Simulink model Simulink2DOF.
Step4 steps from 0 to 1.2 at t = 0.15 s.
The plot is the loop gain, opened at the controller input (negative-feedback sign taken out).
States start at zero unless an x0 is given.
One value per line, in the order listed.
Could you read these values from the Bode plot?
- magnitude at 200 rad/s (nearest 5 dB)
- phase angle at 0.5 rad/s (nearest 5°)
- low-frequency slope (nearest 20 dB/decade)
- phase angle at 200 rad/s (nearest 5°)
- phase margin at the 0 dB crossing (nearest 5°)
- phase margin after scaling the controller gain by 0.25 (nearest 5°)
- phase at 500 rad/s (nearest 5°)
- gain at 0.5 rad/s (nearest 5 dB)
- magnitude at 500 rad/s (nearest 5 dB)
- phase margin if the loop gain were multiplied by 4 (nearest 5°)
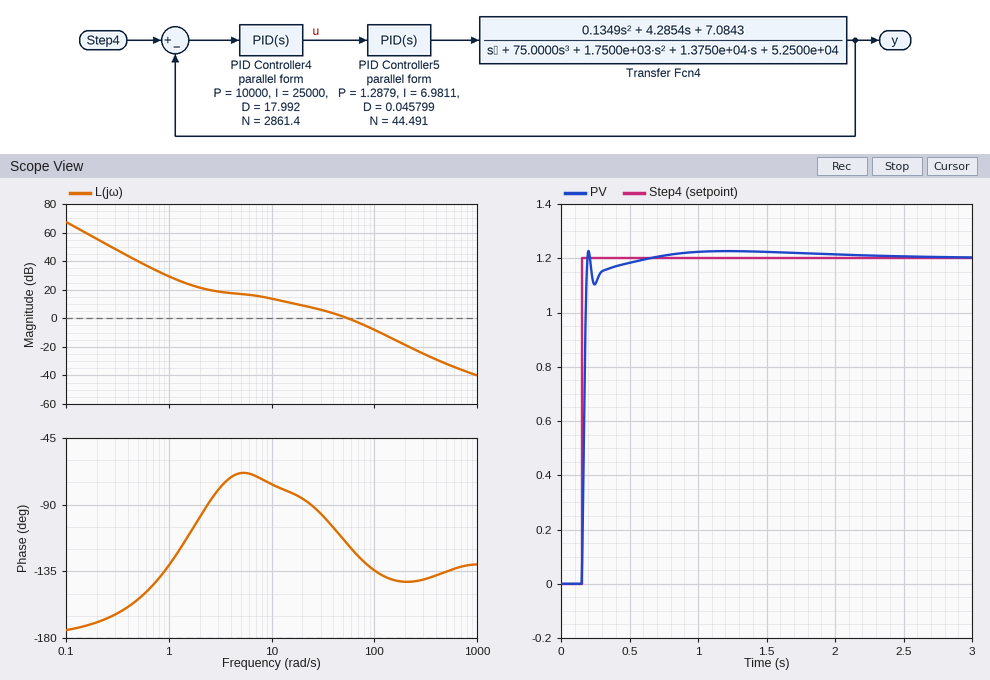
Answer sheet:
-20 dB
-155°
-40 dB/decade
-140°
65°
100°
-135°
40 dB
-30 dB
40°
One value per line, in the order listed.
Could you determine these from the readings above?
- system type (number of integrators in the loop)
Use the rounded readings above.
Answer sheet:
2
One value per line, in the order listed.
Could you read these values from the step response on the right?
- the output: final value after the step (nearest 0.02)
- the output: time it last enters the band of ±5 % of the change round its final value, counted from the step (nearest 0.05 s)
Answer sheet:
1.20
0.15 s
